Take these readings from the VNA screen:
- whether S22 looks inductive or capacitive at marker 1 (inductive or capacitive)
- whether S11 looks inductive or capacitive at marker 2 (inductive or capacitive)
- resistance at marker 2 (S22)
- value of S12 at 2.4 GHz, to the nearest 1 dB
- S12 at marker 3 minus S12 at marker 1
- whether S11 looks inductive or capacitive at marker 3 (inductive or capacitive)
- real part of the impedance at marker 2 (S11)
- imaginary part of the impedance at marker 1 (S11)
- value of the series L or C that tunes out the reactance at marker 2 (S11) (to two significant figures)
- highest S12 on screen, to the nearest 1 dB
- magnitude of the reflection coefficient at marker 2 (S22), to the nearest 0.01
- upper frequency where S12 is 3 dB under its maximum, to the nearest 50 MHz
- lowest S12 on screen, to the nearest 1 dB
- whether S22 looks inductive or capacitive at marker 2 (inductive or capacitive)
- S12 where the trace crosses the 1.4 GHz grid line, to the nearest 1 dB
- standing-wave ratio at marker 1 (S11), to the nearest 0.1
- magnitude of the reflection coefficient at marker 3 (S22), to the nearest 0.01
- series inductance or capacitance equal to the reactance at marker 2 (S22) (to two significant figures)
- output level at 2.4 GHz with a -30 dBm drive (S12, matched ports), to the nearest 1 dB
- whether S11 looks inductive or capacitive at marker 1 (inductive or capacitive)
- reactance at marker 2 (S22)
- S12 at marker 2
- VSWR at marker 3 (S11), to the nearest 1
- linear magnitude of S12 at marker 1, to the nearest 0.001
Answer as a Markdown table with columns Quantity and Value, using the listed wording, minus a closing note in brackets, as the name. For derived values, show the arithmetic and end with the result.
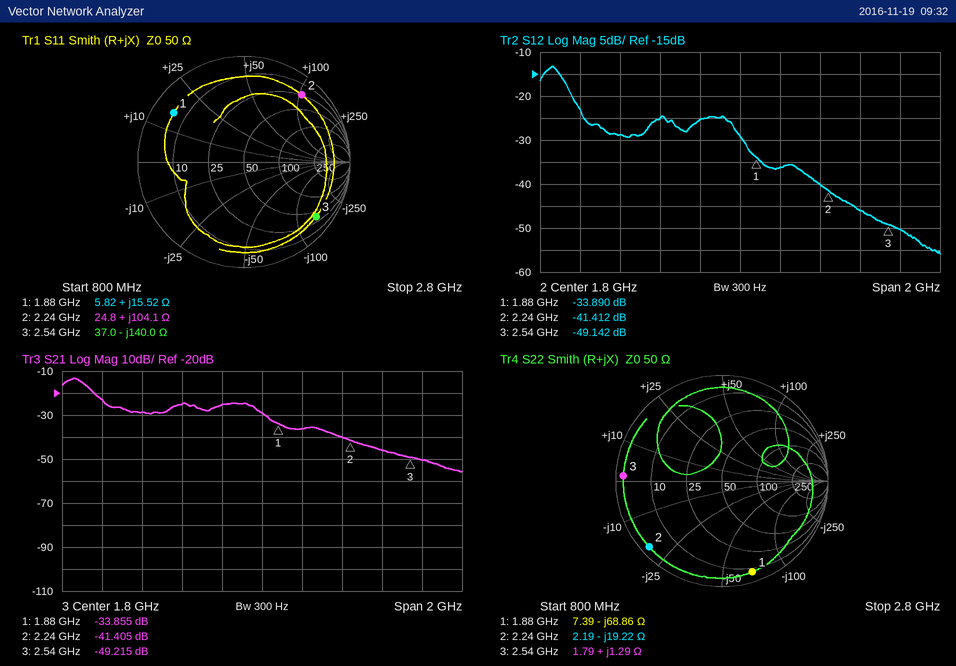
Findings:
| Quantity | Value |
|---|---|
| whether S22 looks inductive or capacitive at marker 1 | capacitive |
| whether S11 looks inductive or capacitive at marker 2 | inductive |
| resistance at marker 2 | 2.19 Ω |
| value of S12 at 2.4 GHz, to the nearest 1 dB | -46 dB |
| S12 at marker 3 minus S12 at marker 1 | -49.142 − (-33.89) = -15.252 dB |
| whether S11 looks inductive or capacitive at marker 3 | capacitive |
| real part of the impedance at marker 2 | 24.8 Ω |
| imaginary part of the impedance at marker 1 | +15.52 Ω |
| value of the series L or C that tunes out the reactance at marker 2 (S11) | C = 1/(2π × 2.24 GHz × 104.1 Ω) ≈ 683 fF, so 680 fF to two significant figures |
| highest S12 on screen, to the nearest 1 dB | -13 dB |
| magnitude of the reflection coefficient at marker 2 (S22), to the nearest 0.01 | 0.93 |
| upper frequency where S12 is 3 dB under its maximum, to the nearest 50 MHz | 900 MHz |
| lowest S12 on screen, to the nearest 1 dB | -56 dB |
| whether S22 looks inductive or capacitive at marker 2 | capacitive |
| S12 where the trace crosses the 1.4 GHz grid line, to the nearest 1 dB | -25 dB |
| standing-wave ratio at marker 1 (S11), to the nearest 0.1 | 9.4 |
| magnitude of the reflection coefficient at marker 3 (S22), to the nearest 0.01 | 0.93 |
| series inductance or capacitance equal to the reactance at marker 2 (S22) | C = 1/(2π × 2.24 GHz × 19.22 Ω) ≈ 3.7 pF |
| output level at 2.4 GHz with a -30 dBm drive (S12, matched ports), to the nearest 1 dB | -30 dBm + (-46 dB) = -76 dBm |
| whether S11 looks inductive or capacitive at marker 1 | inductive |
| reactance at marker 2 | -19.22 Ω |
| S12 at marker 2 | -41.412 dB |
| VSWR at marker 3 (S11), to the nearest 1 | 13 |
| linear magnitude of S12 at marker 1, to the nearest 0.001 | 10^(-33.89/20) ≈ 0.020 |
